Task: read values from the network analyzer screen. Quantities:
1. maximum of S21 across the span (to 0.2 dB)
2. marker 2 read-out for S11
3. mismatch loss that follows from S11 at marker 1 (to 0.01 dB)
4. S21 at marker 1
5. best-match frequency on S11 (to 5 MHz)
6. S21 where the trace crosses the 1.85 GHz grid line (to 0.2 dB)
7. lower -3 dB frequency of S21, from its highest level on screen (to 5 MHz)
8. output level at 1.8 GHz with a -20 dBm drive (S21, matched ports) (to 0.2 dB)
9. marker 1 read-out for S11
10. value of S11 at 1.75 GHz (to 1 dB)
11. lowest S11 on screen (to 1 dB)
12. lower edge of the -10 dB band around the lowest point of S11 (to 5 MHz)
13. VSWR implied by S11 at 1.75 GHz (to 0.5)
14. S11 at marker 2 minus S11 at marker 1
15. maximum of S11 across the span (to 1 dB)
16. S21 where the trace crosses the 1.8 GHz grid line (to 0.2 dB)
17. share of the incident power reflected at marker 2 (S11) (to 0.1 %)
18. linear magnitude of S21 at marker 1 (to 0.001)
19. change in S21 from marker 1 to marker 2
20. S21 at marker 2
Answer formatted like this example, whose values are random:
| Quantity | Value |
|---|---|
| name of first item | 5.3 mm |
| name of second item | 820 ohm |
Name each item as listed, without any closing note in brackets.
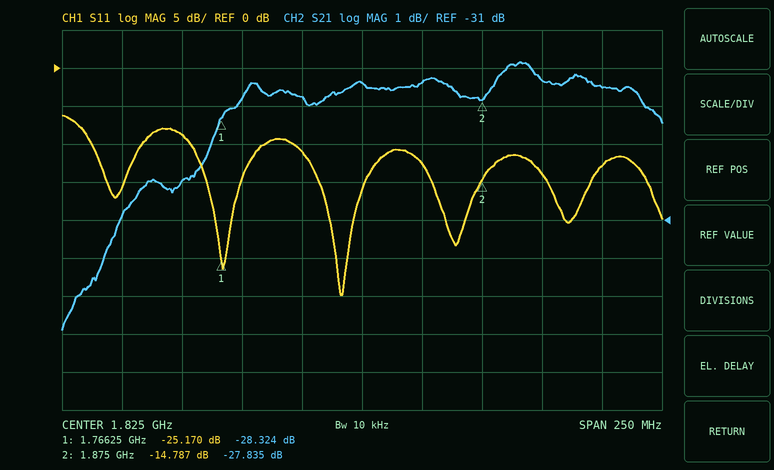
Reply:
| Quantity | Value |
|---|---|
| maximum of S21 across the span | -26.8 dB |
| marker 2 read-out for S11 | -14.787 dB |
| mismatch loss that follows from S11 at marker 1 | 0.01 dB |
| S21 at marker 1 | -28.324 dB |
| best-match frequency on S11 | 1.815 GHz |
| S21 where the trace crosses the 1.85 GHz grid line | -27.4 dB |
| lower -3 dB frequency of S21, from its highest level on screen | 1.755 GHz |
| output level at 1.8 GHz with a -20 dBm drive (S21, matched ports) | -47.8 dBm |
| marker 1 read-out for S11 | -25.170 dB |
| value of S11 at 1.75 GHz | -9 dB |
| lowest S11 on screen | -30 dB |
| lower edge of the -10 dB band around the lowest point of S11 | 1.795 GHz |
| VSWR implied by S11 at 1.75 GHz | 2.0 |
| S11 at marker 2 minus S11 at marker 1 | 10.383 dB |
| maximum of S11 across the span | -6 dB |
| S21 where the trace crosses the 1.8 GHz grid line | -27.8 dB |
| share of the incident power reflected at marker 2 (S11) | 3.3 % |
| linear magnitude of S21 at marker 1 | 0.038 |
| change in S21 from marker 1 to marker 2 | 0.489 dB |
| S21 at marker 2 | -27.835 dB |
